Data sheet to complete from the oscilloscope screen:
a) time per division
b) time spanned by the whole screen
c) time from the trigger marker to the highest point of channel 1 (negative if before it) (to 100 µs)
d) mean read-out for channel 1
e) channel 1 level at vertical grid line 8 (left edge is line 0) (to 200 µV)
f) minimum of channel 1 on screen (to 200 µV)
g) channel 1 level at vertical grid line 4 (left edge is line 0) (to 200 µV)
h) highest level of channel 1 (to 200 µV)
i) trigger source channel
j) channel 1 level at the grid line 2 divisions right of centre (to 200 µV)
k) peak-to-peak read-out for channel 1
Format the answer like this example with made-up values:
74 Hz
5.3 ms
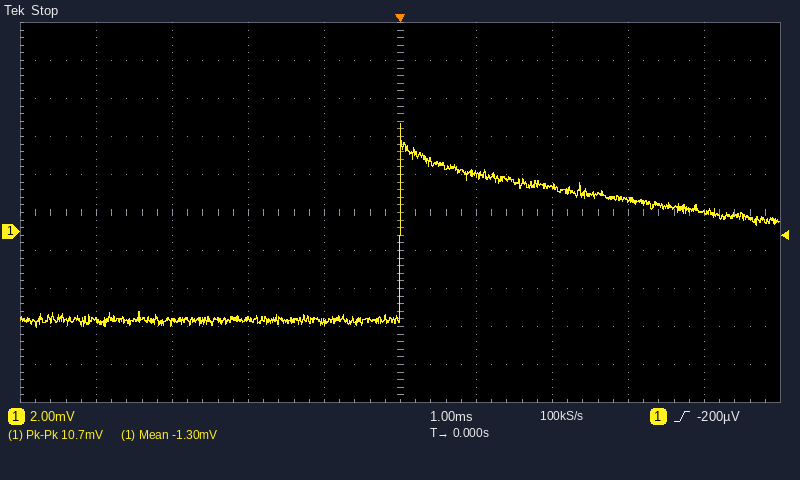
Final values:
1 ms
10 ms
0.0 ms
-1.30 mV
1.6 mV
-5.0 mV
-4.8 mV
5.6 mV
channel 1
2.4 mV
10.7 mV
